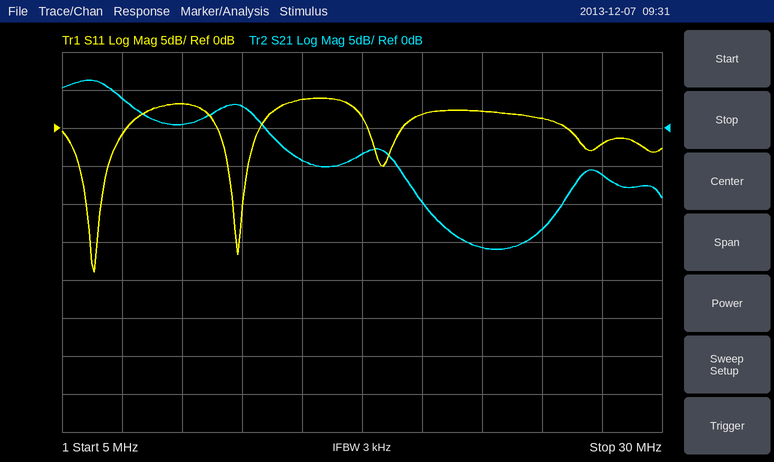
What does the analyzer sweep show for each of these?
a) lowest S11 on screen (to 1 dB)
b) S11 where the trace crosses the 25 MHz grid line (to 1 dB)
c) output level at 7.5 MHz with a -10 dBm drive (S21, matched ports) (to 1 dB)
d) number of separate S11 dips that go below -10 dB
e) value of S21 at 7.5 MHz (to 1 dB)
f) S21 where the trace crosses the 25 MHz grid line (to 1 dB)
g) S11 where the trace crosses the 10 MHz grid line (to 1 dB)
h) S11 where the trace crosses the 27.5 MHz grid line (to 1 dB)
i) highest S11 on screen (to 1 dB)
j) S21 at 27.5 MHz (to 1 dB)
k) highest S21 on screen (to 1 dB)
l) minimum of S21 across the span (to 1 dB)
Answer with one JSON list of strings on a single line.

["-19 dB", "1 dB", "-6 dBm", "2", "4 dB", "-13 dB", "3 dB", "-2 dB", "4 dB", "-6 dB", "6 dB", "-16 dB"]
